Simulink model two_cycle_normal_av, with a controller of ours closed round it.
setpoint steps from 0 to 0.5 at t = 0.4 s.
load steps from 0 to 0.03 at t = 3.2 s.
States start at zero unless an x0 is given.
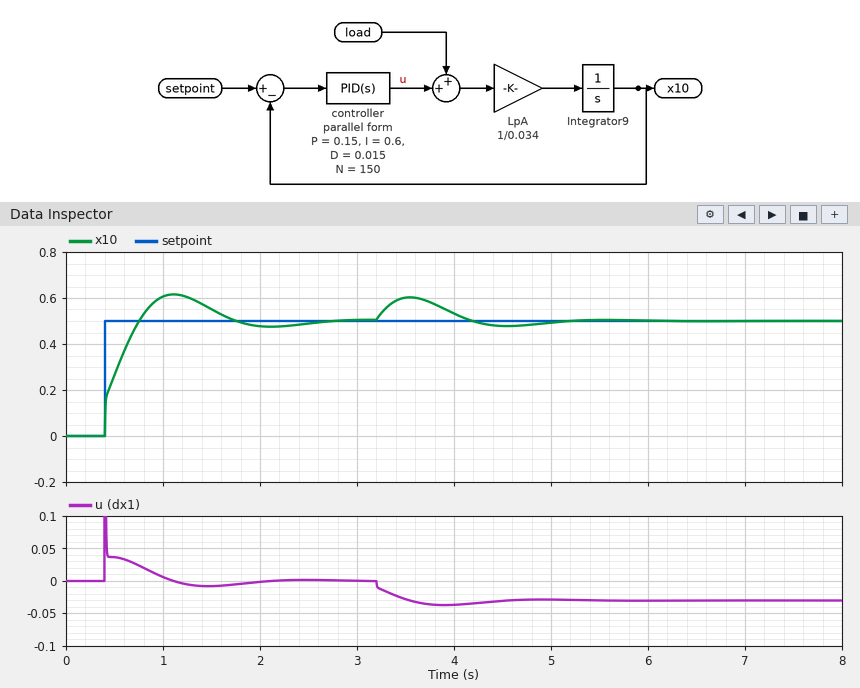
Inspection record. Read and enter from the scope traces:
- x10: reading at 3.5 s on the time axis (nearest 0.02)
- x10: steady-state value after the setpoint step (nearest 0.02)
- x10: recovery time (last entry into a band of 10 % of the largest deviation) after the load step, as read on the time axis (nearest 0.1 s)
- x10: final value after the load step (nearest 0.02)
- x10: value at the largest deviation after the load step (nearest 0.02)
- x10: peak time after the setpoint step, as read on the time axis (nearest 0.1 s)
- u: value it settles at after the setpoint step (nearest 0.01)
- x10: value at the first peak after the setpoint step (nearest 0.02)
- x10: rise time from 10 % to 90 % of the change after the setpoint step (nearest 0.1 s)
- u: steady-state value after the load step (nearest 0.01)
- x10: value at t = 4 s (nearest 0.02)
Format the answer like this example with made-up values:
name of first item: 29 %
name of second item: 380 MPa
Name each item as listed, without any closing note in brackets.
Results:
x10: reading at 3.5 s on the time axis: 0.60
x10: steady-state value after the setpoint step: 0.50
x10: recovery time (last entry into a band of 10 % of the largest deviation) after the load step, as read on the time axis: 4.9 s
x10: final value after the load step: 0.50
x10: value at the largest deviation after the load step: 0.60
x10: peak time after the setpoint step, as read on the time axis: 1.1 s
u: value it settles at after the setpoint step: 0.00
x10: value at the first peak after the setpoint step: 0.62
x10: rise time from 10 % to 90 % of the change after the setpoint step: 0.3 s
u: steady-state value after the load step: -0.03
x10: value at t = 4 s: 0.54
